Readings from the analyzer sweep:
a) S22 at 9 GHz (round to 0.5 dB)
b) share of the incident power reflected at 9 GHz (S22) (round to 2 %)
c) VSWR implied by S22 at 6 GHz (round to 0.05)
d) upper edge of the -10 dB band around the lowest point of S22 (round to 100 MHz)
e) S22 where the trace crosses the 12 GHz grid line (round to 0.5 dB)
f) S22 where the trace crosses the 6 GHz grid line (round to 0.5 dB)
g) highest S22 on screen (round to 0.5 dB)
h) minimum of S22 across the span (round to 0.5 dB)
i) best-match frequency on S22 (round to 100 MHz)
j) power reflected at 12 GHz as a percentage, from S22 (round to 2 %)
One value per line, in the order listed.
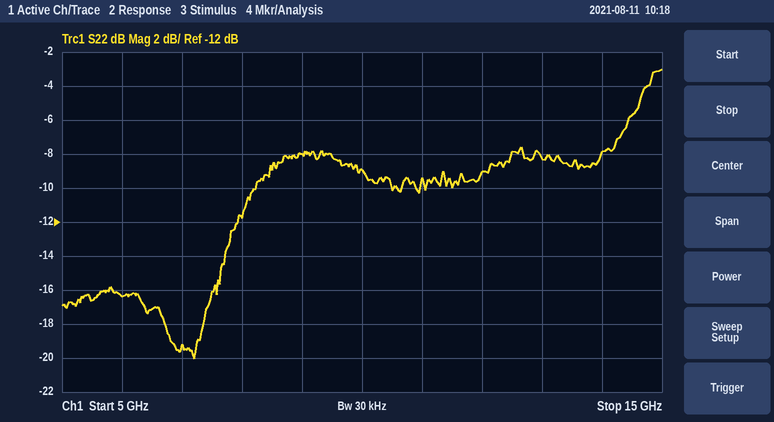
-8.0 dB
16 %
1.35
8.2 GHz
-9.0 dB
-16.5 dB
-3.0 dB
-20.0 dB
7.2 GHz
12 %
